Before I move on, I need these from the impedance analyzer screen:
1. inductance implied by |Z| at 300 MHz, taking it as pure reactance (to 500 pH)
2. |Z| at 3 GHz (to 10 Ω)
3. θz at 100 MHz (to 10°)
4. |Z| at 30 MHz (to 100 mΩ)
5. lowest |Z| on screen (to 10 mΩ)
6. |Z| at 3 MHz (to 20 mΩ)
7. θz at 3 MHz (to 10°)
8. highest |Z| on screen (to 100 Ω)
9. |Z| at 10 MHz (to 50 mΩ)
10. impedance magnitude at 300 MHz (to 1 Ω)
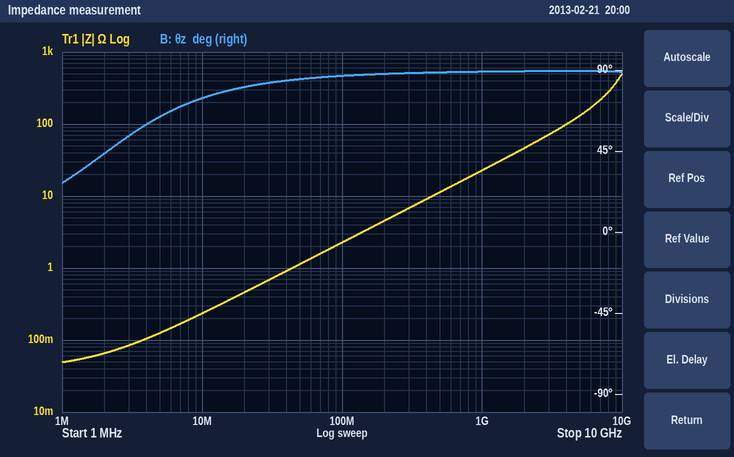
3.5 nH
70 Ω
90°
700 mΩ
50 mΩ
80 mΩ
50°
500 Ω
250 mΩ
7 Ω
